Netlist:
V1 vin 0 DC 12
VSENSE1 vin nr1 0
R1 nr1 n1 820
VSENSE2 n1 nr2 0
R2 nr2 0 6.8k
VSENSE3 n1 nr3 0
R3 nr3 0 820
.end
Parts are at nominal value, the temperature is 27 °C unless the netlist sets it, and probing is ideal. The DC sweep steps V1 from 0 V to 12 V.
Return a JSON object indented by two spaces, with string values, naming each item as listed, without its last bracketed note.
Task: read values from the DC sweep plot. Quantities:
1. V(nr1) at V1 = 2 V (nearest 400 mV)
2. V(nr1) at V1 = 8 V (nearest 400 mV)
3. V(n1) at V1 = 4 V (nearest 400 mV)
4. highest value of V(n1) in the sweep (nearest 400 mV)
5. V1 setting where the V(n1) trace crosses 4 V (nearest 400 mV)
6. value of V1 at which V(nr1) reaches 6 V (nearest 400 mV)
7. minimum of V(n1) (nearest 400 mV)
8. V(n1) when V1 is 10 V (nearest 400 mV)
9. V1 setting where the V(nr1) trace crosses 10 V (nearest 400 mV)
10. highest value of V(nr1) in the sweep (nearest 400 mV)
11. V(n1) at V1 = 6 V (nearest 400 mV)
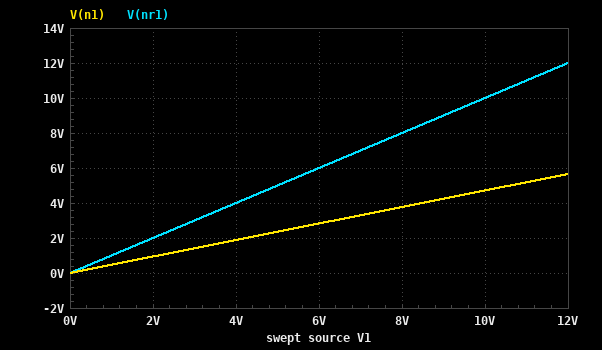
{
  "V(nr1) at V1 = 2 V": "2.0 V",
  "V(nr1) at V1 = 8 V": "8.0 V",
  "V(n1) at V1 = 4 V": "2.0 V",
  "highest value of V(n1) in the sweep": "5.6 V",
  "V1 setting where the V(n1) trace crosses 4 V": "8.4 V",
  "value of V1 at which V(nr1) reaches 6 V": "6.0 V",
  "minimum of V(n1)": "0 V",
  "V(n1) when V1 is 10 V": "4.8 V",
  "V1 setting where the V(nr1) trace crosses 10 V": "10.0 V",
  "highest value of V(nr1) in the sweep": "12.0 V",
  "V(n1) at V1 = 6 V": "2.8 V"
}
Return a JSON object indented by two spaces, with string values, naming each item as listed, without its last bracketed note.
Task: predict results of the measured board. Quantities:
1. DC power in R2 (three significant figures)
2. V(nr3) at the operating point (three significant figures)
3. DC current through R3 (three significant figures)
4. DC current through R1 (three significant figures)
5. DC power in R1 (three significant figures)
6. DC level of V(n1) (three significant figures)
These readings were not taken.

{
  "DC power in R2": "4.71 mW",
  "V(nr3) at the operating point": "5.66 V",
  "DC current through R3": "6.90 mA",
  "DC current through R1": "7.73 mA",
  "DC power in R1": "49.0 mW",
  "DC level of V(n1)": "5.66 V"
}
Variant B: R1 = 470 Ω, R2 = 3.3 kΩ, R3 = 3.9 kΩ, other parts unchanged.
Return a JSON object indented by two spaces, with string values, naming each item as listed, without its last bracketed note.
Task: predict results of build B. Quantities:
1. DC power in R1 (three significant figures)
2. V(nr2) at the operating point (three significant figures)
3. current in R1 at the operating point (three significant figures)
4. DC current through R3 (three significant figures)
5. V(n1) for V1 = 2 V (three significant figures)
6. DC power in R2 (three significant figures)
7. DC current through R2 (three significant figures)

{
  "DC power in R1": "13.3 mW",
  "V(nr2) at the operating point": "9.50 V",
  "current in R1 at the operating point": "5.32 mA",
  "DC current through R3": "2.44 mA",
  "V(n1) for V1 = 2 V": "1.58 V",
  "DC power in R2": "27.4 mW",
  "DC current through R2": "2.88 mA"
}
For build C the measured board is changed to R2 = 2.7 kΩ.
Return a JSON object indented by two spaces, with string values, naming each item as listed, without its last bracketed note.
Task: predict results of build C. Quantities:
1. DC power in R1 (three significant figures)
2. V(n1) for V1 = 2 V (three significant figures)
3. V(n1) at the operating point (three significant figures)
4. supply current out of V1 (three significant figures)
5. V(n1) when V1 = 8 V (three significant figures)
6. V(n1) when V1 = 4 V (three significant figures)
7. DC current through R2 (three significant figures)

{
  "DC power in R1": "56.2 mW",
  "V(n1) for V1 = 2 V": "868 mV",
  "V(n1) at the operating point": "5.21 V",
  "supply current out of V1": "8.28 mA",
  "V(n1) when V1 = 8 V": "3.47 V",
  "V(n1) when V1 = 4 V": "1.74 V",
  "DC current through R2": "1.93 mA"
}
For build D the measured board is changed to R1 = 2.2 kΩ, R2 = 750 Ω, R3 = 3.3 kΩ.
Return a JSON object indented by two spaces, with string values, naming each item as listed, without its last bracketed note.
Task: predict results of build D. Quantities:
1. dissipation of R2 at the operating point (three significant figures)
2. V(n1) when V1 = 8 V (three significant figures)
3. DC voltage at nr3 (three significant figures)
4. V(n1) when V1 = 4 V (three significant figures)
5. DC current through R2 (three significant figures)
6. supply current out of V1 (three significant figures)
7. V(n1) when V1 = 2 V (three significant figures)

{
  "dissipation of R2 at the operating point": "9.07 mW",
  "V(n1) when V1 = 8 V": "1.74 V",
  "DC voltage at nr3": "2.61 V",
  "V(n1) when V1 = 4 V": "870 mV",
  "DC current through R2": "3.48 mA",
  "supply current out of V1": "4.27 mA",
  "V(n1) when V1 = 2 V": "435 mV"
}
